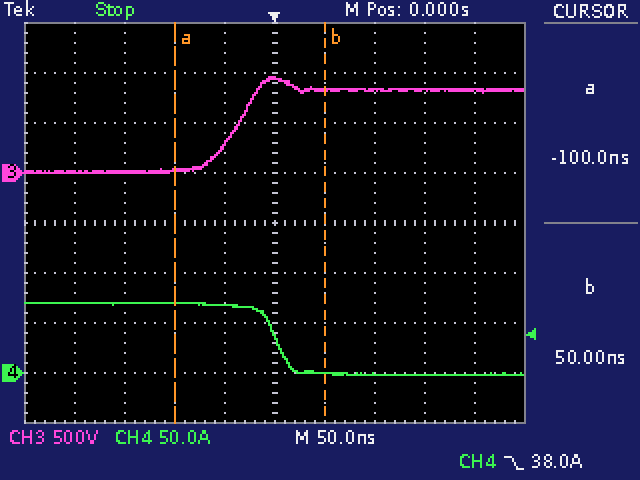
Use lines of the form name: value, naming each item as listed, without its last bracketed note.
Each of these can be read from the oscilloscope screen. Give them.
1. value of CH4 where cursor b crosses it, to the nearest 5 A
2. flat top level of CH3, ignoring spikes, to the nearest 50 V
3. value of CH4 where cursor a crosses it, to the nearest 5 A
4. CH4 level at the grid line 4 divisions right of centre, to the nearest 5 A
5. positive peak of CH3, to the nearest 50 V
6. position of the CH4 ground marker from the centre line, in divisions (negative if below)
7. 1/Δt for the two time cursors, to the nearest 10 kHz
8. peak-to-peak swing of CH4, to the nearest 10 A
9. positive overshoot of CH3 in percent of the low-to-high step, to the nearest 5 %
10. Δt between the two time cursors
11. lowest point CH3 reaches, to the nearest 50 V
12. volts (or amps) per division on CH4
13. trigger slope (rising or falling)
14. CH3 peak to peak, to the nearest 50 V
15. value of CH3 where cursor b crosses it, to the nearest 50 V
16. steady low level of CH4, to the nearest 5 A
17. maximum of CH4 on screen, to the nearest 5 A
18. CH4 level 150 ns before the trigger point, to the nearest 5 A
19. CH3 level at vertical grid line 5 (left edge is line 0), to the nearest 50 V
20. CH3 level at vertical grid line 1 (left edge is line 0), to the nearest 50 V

value of CH4 where cursor b crosses it, to the nearest 5 A: 0 A
flat top level of CH3, ignoring spikes, to the nearest 50 V: 850 V
value of CH4 where cursor a crosses it, to the nearest 5 A: 70 A
CH4 level at the grid line 4 divisions right of centre, to the nearest 5 A: 0 A
positive peak of CH3, to the nearest 50 V: 950 V
position of the CH4 ground marker from the centre line, in divisions: -3.0 div
1/Δt for the two time cursors, to the nearest 10 kHz: 6.67 MHz
peak-to-peak swing of CH4, to the nearest 10 A: 70 A
positive overshoot of CH3 in percent of the low-to-high step, to the nearest 5 %: 15 %
Δt between the two time cursors: 150 ns
lowest point CH3 reaches, to the nearest 50 V: 0 V
volts (or amps) per division on CH4: 50 A
trigger slope: falling
CH3 peak to peak, to the nearest 50 V: 950 V
value of CH3 where cursor b crosses it, to the nearest 50 V: 850 V
steady low level of CH4, to the nearest 5 A: 0 A
maximum of CH4 on screen, to the nearest 5 A: 70 A
CH4 level 150 ns before the trigger point, to the nearest 5 A: 70 A
CH3 level at vertical grid line 5 (left edge is line 0), to the nearest 50 V: 950 V
CH3 level at vertical grid line 1 (left edge is line 0), to the nearest 50 V: 0 V
